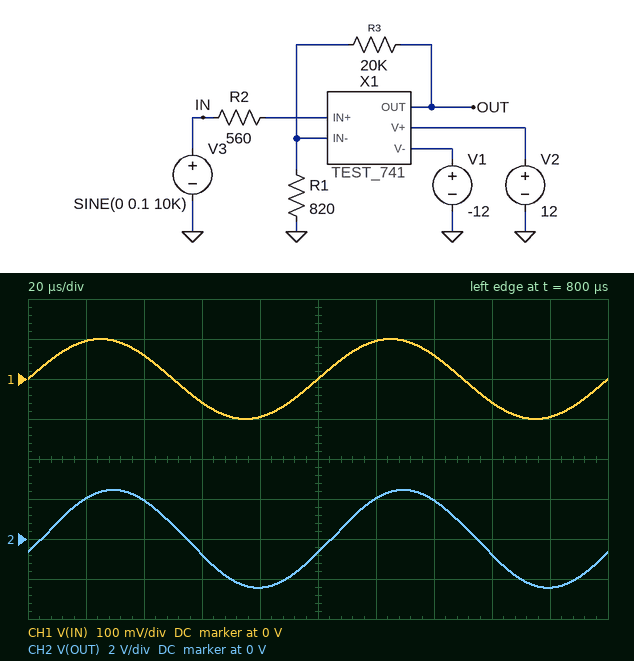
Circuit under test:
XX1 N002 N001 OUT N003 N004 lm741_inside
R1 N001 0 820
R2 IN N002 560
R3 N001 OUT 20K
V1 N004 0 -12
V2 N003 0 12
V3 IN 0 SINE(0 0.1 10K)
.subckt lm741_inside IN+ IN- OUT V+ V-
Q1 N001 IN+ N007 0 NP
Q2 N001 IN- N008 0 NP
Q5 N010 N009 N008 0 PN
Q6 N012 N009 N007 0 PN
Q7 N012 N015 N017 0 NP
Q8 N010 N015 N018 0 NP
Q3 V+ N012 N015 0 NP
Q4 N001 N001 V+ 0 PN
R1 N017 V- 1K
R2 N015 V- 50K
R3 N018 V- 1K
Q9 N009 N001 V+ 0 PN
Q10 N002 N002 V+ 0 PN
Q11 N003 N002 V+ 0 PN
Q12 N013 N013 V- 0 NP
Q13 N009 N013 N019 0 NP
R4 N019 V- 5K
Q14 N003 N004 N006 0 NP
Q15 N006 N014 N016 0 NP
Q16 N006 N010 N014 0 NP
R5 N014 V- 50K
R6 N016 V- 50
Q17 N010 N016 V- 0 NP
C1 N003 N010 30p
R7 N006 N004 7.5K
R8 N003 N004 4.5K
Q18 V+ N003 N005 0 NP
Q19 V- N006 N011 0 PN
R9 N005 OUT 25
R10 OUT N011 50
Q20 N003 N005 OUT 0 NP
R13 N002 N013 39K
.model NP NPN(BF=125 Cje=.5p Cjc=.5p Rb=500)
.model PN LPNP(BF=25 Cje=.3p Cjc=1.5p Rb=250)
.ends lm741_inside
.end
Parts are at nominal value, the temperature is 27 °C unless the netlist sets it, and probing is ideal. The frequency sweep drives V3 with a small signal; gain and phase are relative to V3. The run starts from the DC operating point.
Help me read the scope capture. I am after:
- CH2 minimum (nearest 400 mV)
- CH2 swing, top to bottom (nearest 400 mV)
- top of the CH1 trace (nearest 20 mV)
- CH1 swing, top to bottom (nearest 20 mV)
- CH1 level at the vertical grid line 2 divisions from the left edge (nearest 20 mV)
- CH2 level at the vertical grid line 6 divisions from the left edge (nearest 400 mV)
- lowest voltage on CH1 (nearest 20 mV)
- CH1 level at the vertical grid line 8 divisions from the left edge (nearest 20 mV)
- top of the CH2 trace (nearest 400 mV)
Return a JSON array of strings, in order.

["-2.4 V", "4.8 V", "100 mV", "200 mV", "60 mV", "2.0 V", "-100 mV", "-60 mV", "2.4 V"]
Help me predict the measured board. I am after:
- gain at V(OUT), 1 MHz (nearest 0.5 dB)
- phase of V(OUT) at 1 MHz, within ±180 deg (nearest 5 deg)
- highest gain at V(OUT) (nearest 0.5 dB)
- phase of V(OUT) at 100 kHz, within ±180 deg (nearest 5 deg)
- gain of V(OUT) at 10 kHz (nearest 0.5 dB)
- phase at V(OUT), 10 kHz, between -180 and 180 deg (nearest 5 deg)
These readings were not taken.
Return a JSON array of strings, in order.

["-3.0 dB", "-90 deg", "28.0 dB", "-75 deg", "27.5 dB", "-20 deg"]
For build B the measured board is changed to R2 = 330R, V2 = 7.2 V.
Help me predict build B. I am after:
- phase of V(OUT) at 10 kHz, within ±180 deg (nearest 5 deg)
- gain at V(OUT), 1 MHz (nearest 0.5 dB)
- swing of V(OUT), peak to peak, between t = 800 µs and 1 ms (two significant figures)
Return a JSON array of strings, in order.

["-25 deg", "-4.5 dB", "4.9 V"]
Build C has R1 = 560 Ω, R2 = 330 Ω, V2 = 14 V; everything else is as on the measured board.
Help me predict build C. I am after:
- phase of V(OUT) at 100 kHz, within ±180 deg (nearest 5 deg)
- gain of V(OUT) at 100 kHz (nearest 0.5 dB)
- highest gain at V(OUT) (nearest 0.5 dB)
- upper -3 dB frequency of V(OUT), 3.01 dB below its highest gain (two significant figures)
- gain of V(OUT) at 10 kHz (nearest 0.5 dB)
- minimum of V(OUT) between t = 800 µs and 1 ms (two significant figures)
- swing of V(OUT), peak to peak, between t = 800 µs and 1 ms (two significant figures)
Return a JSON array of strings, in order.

["-80 deg", "17.0 dB", "31.5 dB", "20 kHz", "30.5 dB", "-3.4 V", "6.8 V"]
